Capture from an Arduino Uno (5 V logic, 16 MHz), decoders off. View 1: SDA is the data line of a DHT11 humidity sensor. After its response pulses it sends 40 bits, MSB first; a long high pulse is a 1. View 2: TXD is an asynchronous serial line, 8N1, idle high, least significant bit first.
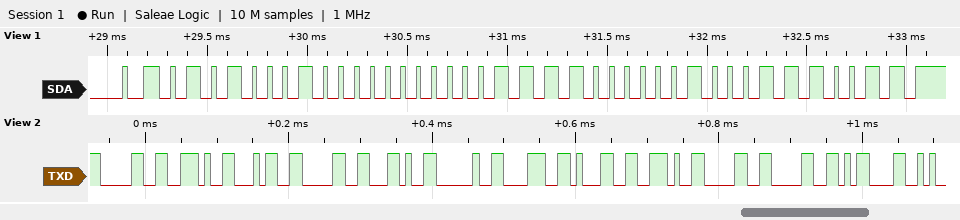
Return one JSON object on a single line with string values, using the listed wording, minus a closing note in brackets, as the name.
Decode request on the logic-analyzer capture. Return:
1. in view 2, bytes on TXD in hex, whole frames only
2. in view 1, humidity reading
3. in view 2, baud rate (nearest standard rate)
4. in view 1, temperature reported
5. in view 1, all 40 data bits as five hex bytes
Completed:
{"in view 2, bytes on TXD in hex, whole frames only": "30 2E 34 30 2C 20 38 31 2E 30 30 0D", "in view 1, humidity reading": "81 %", "in view 2, baud rate": "115200 baud", "in view 1, temperature reported": "30.4 °C", "in view 1, all 40 data bits as five hex bytes": "51 00 1E 04 73"}
